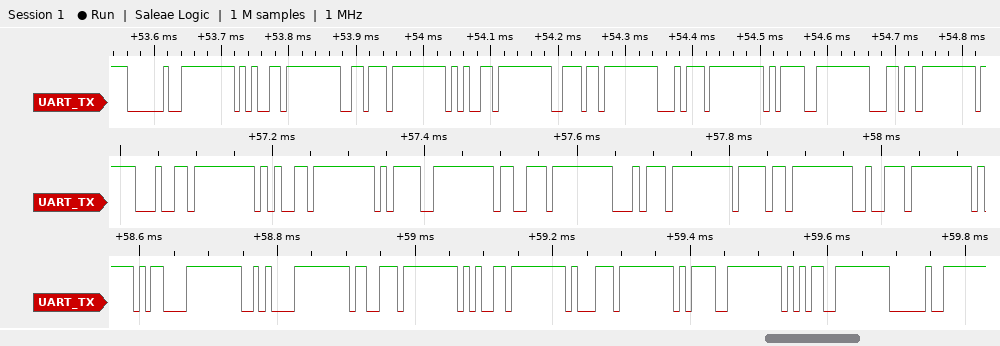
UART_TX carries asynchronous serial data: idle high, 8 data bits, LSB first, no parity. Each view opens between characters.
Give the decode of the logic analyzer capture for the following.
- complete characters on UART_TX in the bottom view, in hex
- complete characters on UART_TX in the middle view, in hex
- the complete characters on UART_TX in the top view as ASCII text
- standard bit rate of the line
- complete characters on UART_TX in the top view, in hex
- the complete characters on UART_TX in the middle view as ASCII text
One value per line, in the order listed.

0D, 0A, 73, 65, 71, 3D, 35, 20
64, 65, 3D, 73, 74, 6F, 72
" event=l"
115200 baud
20, 65, 76, 65, 6E, 74, 3D, 6C
"de=stor"
